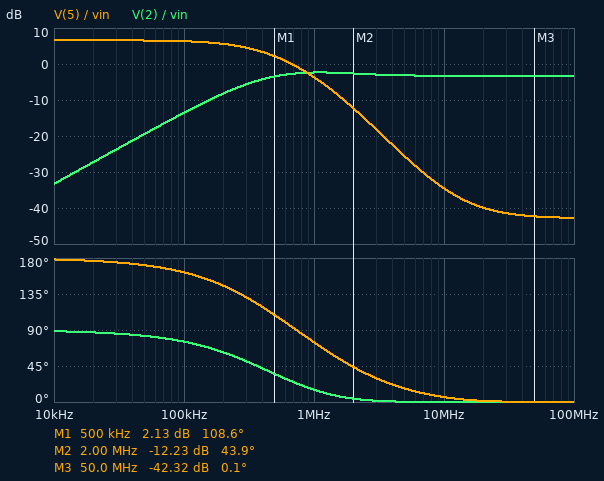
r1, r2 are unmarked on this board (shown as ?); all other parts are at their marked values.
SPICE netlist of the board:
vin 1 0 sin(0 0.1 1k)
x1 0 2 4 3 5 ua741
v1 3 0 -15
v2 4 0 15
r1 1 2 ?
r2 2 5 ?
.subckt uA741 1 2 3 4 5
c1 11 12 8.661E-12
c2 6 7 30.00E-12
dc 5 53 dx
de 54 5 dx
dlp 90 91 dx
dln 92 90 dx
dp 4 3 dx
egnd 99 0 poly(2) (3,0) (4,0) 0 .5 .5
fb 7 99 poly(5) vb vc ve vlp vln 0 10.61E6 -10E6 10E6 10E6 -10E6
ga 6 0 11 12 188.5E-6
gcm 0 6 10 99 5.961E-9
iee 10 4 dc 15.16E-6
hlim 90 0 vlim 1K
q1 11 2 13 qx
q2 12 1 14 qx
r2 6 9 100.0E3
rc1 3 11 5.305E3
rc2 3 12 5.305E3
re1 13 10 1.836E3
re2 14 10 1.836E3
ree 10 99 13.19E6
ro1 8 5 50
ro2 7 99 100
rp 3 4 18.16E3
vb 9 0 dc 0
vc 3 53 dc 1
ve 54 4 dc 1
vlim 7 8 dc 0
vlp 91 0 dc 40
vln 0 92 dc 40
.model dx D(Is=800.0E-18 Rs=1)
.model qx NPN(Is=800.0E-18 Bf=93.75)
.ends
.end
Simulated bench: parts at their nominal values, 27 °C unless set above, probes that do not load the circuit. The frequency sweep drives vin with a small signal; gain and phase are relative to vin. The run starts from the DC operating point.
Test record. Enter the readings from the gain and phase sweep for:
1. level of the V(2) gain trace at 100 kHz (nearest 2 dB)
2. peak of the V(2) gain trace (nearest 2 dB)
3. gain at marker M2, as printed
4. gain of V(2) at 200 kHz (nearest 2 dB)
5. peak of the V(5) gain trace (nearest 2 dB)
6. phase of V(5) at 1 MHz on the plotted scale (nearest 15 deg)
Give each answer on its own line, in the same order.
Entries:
-14 dB
-2 dB
-12.23 dB
-8 dB
6 dB
75 deg
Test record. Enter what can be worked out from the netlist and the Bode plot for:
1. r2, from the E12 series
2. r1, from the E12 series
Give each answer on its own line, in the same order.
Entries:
4.7 kΩ
2.2 kΩ
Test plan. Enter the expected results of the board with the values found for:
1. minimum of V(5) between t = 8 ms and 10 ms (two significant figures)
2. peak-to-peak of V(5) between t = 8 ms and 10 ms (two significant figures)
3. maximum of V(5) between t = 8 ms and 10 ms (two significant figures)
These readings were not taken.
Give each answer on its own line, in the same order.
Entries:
-210 mV
430 mV
210 mV
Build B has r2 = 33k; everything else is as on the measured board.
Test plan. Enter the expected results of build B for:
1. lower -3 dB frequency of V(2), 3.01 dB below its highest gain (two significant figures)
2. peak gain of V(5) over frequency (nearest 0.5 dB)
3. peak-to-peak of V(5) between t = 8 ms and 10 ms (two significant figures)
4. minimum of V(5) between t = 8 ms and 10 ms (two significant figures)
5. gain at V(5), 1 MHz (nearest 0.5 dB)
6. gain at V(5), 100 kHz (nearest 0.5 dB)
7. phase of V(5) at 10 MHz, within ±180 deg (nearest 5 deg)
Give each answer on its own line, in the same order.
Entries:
63 kHz
23.5 dB
3.0 V
-1.5 V
-1.5 dB
18.0 dB
10 deg
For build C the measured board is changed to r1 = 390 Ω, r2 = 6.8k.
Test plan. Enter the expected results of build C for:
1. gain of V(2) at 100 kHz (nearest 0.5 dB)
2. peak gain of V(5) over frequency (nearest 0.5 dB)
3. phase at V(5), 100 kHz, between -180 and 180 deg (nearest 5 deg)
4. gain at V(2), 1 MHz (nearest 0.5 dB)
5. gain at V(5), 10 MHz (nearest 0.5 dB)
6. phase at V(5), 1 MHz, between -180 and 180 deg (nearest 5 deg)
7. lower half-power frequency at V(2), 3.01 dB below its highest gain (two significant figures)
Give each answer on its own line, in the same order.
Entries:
-1.5 dB
25.0 dB
115 deg
-0.5 dB
-33.0 dB
60 deg
55 kHz
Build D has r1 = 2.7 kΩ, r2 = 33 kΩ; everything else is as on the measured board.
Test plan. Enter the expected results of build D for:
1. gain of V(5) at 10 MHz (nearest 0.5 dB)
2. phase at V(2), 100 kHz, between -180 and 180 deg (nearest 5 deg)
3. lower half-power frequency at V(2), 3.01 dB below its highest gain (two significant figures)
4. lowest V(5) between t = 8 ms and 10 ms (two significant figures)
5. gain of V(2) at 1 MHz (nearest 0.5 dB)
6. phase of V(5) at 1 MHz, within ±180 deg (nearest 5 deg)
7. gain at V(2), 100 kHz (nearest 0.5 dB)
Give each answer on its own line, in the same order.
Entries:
-35.5 dB
40 deg
77 kHz
-1.2 V
-0.5 dB
65 deg
-2.5 dB
